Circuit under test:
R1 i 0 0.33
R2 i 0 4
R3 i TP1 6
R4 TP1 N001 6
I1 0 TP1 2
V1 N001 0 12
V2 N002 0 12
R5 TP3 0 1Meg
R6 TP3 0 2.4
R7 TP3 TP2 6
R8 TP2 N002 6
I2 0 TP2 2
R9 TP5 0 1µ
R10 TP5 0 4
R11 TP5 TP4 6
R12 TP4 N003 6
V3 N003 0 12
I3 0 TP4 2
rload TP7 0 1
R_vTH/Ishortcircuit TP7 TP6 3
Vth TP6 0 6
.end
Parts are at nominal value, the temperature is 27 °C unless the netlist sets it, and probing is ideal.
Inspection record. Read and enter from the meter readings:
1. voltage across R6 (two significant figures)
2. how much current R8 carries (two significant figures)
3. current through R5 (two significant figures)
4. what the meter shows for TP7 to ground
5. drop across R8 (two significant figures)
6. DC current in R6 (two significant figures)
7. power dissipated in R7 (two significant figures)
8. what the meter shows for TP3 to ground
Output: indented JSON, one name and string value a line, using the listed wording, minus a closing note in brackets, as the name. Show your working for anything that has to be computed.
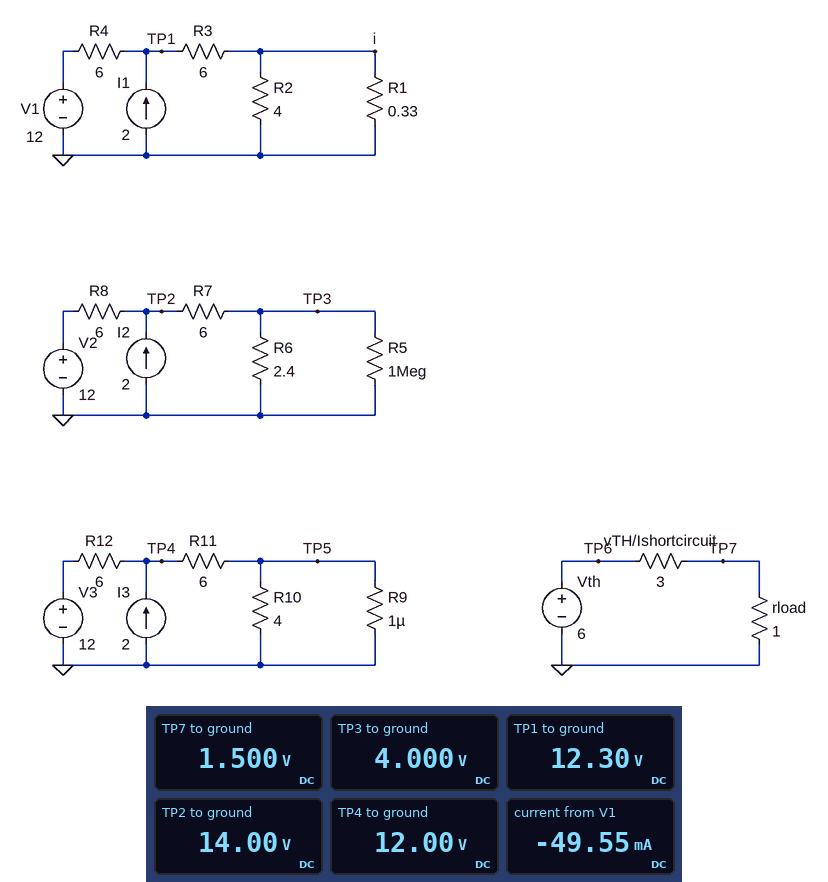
{
  "voltage across R6": "4 V = 4.0 V",
  "how much current R8 carries": "(14 V - 12 V) / 6 Ω = 330 mA",
  "current through R5": "(4 V) / 1 MΩ = 4.0 µA",
  "what the meter shows for TP7 to ground": "1.500 V",
  "drop across R8": "14 V - 12 V = 2.0 V",
  "DC current in R6": "(4 V) / 2.4 Ω = 1.7 A",
  "power dissipated in R7": "(14 V - 4 V)^2 / 6 Ω = 17 W",
  "what the meter shows for TP3 to ground": "4.000 V"
}
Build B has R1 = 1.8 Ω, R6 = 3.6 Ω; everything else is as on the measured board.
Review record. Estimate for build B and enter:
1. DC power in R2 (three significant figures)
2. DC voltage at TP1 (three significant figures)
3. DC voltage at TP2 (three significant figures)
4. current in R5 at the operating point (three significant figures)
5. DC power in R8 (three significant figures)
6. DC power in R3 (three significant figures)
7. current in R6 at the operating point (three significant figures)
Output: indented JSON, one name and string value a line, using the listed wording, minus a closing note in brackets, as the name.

{
  "DC power in R2": "1.27 W",
  "DC voltage at TP1": "13.1 V",
  "DC voltage at TP2": "14.8 V",
  "current in R5 at the operating point": "5.54 µA",
  "DC power in R8": "1.28 W",
  "DC power in R3": "19.7 W",
  "current in R6 at the operating point": "1.54 A"
}
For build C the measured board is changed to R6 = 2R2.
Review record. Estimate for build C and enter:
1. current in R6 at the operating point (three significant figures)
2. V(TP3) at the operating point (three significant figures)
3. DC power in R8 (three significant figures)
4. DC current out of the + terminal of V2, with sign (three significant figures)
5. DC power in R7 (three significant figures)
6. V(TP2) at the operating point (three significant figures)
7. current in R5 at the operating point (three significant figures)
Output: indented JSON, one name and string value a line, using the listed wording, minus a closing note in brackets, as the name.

{
  "current in R6 at the operating point": "1.69 A",
  "V(TP3) at the operating point": "3.72 V",
  "DC power in R8": "576 mW",
  "DC current out of the + terminal of V2, with sign": "-310 mA",
  "DC power in R7": "17.1 W",
  "V(TP2) at the operating point": "13.9 V",
  "current in R5 at the operating point": "3.72 µA"
}
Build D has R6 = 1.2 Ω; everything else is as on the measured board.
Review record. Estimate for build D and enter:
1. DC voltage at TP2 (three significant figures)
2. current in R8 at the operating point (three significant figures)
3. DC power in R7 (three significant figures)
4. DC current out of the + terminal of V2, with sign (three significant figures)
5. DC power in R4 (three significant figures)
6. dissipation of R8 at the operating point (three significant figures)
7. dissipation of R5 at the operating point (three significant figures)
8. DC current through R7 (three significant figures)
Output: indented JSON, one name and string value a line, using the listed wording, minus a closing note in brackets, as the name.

{
  "DC voltage at TP2": "13.1 V",
  "current in R8 at the operating point": "182 mA",
  "DC power in R7": "19.8 W",
  "DC current out of the + terminal of V2, with sign": "-182 mA",
  "DC power in R4": "14.7 mW",
  "dissipation of R8 at the operating point": "198 mW",
  "dissipation of R5 at the operating point": "4.76 µW",
  "DC current through R7": "1.82 A"
}
